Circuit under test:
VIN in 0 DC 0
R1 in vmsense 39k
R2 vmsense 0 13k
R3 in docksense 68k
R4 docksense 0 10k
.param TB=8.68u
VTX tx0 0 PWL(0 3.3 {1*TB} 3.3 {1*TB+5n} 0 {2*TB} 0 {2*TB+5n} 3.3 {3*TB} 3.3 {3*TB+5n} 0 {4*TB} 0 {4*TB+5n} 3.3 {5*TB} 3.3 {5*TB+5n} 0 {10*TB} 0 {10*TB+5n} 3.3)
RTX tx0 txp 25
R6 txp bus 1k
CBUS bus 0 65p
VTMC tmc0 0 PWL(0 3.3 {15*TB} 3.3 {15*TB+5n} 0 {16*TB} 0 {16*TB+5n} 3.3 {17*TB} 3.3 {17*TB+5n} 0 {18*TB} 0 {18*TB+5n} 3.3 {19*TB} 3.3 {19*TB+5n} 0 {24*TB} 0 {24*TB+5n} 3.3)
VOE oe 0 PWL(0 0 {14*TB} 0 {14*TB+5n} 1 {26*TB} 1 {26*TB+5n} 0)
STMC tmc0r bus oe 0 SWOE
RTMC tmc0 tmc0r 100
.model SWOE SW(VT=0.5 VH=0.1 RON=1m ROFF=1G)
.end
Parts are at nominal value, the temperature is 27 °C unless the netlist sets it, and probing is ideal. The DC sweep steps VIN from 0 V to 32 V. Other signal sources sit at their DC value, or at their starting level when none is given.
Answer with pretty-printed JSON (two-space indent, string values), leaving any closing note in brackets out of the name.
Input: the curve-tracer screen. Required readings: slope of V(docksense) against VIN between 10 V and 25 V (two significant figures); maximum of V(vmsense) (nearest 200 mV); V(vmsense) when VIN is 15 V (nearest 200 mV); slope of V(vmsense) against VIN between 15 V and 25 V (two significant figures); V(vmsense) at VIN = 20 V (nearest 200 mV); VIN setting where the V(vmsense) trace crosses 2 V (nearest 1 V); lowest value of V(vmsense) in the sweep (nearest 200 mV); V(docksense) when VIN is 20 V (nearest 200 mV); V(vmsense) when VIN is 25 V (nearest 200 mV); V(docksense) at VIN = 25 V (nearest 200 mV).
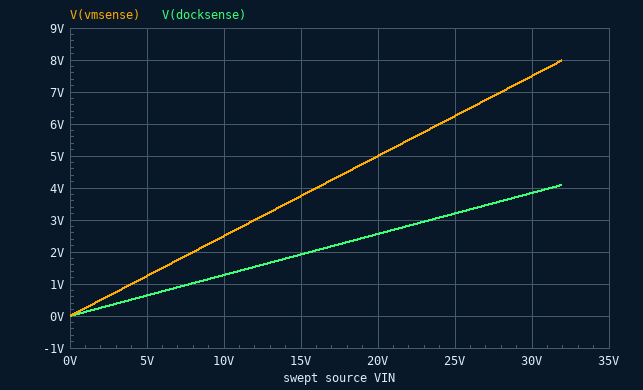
{
  "slope of V(docksense) against VIN between 10 V and 25 V": "0.13 V/V",
  "maximum of V(vmsense)": "8.0 V",
  "V(vmsense) when VIN is 15 V": "3.8 V",
  "slope of V(vmsense) against VIN between 15 V and 25 V": "0.25 V/V",
  "V(vmsense) at VIN = 20 V": "5.0 V",
  "VIN setting where the V(vmsense) trace crosses 2 V": "8 V",
  "lowest value of V(vmsense) in the sweep": "0 V",
  "V(docksense) when VIN is 20 V": "2.6 V",
  "V(vmsense) when VIN is 25 V": "6.2 V",
  "V(docksense) at VIN = 25 V": "3.2 V"
}
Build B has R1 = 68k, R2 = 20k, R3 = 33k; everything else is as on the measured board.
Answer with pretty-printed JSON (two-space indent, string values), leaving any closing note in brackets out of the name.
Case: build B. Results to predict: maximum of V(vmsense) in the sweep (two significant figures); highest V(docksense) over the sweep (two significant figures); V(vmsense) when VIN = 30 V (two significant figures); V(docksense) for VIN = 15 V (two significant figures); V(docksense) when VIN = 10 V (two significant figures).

{
  "maximum of V(vmsense) in the sweep": "7.3 V",
  "highest V(docksense) over the sweep": "7.4 V",
  "V(vmsense) when VIN = 30 V": "6.8 V",
  "V(docksense) for VIN = 15 V": "3.5 V",
  "V(docksense) when VIN = 10 V": "2.3 V"
}
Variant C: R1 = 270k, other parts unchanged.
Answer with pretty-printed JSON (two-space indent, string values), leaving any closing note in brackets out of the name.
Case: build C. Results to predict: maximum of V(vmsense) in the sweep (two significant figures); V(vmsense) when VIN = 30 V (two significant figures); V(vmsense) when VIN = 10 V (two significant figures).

{
  "maximum of V(vmsense) in the sweep": "1.5 V",
  "V(vmsense) when VIN = 30 V": "1.4 V",
  "V(vmsense) when VIN = 10 V": "460 mV"
}
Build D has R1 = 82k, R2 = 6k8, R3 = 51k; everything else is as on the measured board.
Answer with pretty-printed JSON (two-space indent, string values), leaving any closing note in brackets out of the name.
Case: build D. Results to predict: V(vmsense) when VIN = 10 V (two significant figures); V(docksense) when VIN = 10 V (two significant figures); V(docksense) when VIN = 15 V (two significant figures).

{
  "V(vmsense) when VIN = 10 V": "770 mV",
  "V(docksense) when VIN = 10 V": "1.6 V",
  "V(docksense) when VIN = 15 V": "2.5 V"
}
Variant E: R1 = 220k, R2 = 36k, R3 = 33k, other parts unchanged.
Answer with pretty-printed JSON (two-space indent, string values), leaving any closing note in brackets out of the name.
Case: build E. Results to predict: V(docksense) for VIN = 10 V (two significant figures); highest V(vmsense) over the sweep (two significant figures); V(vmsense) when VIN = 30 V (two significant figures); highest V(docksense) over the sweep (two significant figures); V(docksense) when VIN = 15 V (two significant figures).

{
  "V(docksense) for VIN = 10 V": "2.3 V",
  "highest V(vmsense) over the sweep": "4.5 V",
  "V(vmsense) when VIN = 30 V": "4.2 V",
  "highest V(docksense) over the sweep": "7.4 V",
  "V(docksense) when VIN = 15 V": "3.5 V"
}
